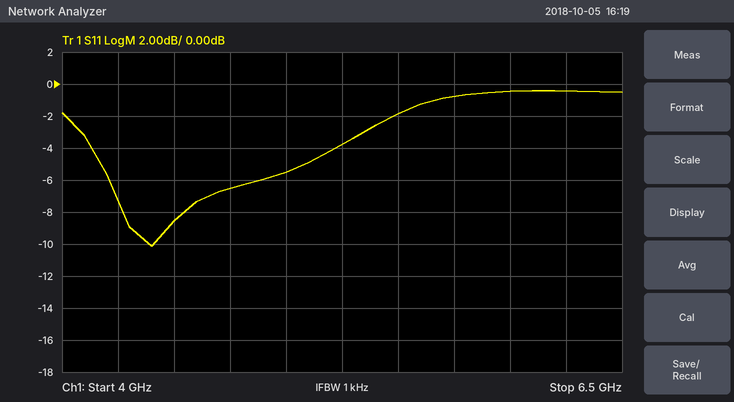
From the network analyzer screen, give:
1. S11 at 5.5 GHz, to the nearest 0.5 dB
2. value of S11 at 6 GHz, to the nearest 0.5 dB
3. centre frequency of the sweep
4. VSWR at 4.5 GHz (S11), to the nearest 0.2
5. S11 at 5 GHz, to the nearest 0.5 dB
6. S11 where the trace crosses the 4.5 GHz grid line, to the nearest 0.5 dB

-2.0 dB
-0.5 dB
5.25 GHz
2.2
-5.5 dB
-8.5 dB
